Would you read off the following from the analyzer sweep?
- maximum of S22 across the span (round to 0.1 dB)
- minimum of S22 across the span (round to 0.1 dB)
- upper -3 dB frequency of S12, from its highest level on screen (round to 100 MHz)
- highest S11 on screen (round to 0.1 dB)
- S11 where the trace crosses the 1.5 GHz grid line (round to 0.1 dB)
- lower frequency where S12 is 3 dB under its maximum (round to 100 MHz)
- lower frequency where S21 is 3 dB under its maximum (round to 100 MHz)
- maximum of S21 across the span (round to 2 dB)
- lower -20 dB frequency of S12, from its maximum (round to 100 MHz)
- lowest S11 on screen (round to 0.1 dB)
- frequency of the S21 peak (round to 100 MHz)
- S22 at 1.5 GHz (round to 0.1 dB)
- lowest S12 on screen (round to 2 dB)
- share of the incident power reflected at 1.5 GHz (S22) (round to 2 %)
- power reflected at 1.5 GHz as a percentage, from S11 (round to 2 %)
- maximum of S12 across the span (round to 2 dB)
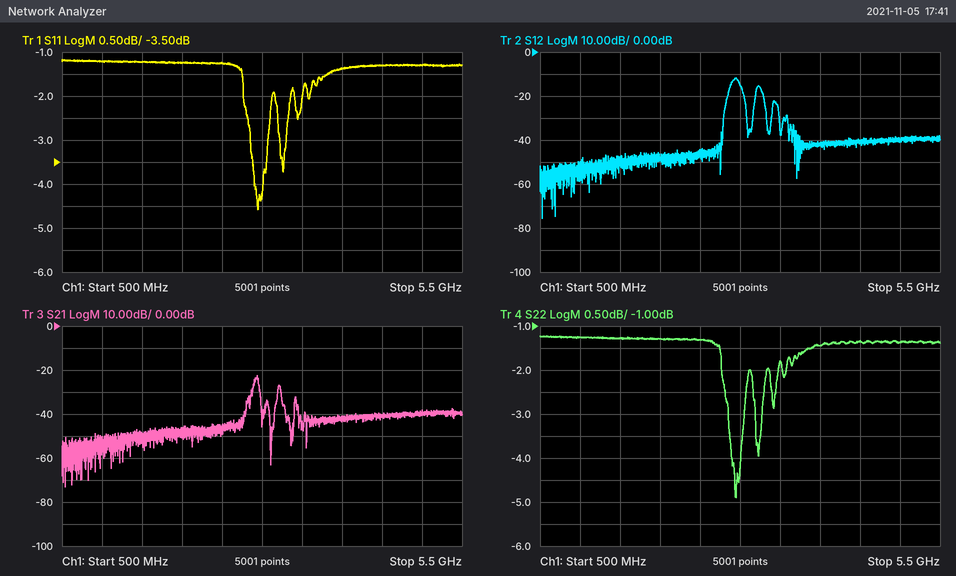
-1.2 dB
-4.9 dB
3.0 GHz
-1.2 dB
-1.2 dB
2.9 GHz
2.9 GHz
-22 dB
2.8 GHz
-4.6 dB
2.9 GHz
-1.3 dB
-76 dB
74 %
76 %
-12 dB
